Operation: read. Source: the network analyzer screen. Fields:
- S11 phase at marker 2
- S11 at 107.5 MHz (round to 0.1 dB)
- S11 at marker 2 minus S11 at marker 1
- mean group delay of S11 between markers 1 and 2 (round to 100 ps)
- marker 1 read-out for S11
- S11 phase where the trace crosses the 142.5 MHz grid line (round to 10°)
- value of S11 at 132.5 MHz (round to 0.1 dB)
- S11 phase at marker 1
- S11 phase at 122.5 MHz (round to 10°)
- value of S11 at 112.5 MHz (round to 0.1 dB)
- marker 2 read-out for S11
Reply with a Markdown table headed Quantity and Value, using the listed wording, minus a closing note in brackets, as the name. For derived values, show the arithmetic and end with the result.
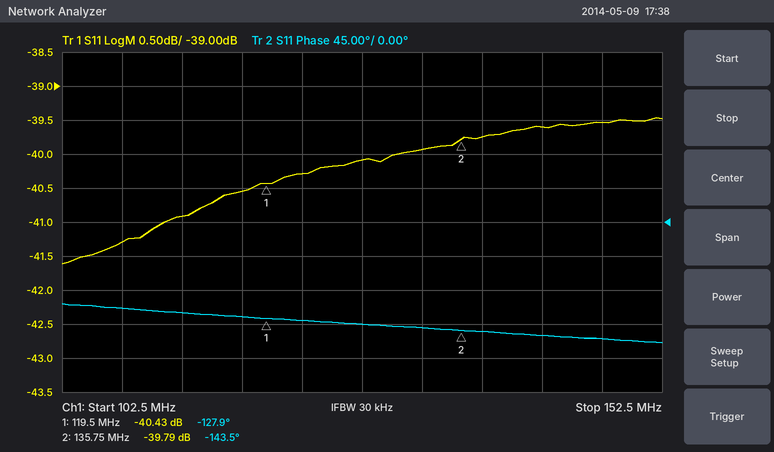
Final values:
| Quantity | Value |
|---|---|
| S11 phase at marker 2 | -143.5° |
| S11 at 107.5 MHz | -41.3 dB |
| S11 at marker 2 minus S11 at marker 1 | -39.79 − (-40.43) = 0.64 dB |
| mean group delay of S11 between markers 1 and 2 | −(-143.5° − (-127.9°))/(360° × 16.25 MHz) ≈ 2.7 ns |
| marker 1 read-out for S11 | -40.43 dB |
| S11 phase where the trace crosses the 142.5 MHz grid line | -150° |
| value of S11 at 132.5 MHz | -39.9 dB |
| S11 phase at marker 1 | -127.9° |
| S11 phase at 122.5 MHz | -130° |
| value of S11 at 112.5 MHz | -40.9 dB |
| marker 2 read-out for S11 | -39.79 dB |
